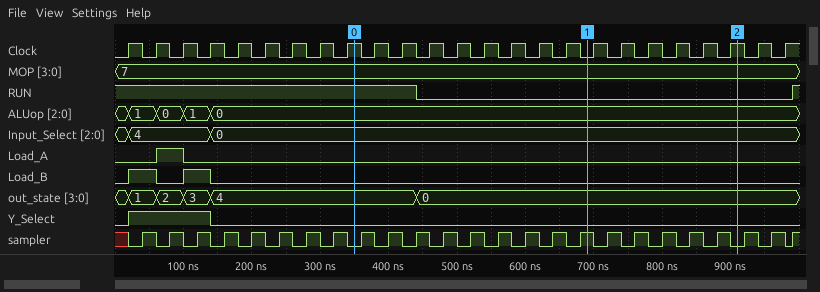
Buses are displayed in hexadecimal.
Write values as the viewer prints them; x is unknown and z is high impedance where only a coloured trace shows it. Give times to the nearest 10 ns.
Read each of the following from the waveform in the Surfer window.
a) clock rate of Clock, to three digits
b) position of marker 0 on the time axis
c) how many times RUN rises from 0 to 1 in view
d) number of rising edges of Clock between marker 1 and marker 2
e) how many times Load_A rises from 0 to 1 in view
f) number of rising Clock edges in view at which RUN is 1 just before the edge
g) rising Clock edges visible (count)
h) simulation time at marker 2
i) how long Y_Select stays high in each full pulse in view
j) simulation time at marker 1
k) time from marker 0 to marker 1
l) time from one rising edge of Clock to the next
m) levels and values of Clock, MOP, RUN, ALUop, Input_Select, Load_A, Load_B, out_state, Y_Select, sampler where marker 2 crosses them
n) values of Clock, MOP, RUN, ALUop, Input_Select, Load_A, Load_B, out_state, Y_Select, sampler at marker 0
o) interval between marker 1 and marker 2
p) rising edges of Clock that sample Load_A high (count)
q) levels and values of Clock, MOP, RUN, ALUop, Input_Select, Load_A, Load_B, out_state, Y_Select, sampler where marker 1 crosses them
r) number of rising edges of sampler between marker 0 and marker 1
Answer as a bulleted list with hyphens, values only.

- 25.0 MHz
- 350 ns
- 1
- 6
- 1
- 11
- 25
- 910 ns
- 120 ns
- 690 ns
- 340 ns
- 40 ns
- Clock=1, MOP=7, RUN=0, ALUop=0, Input_Select=0, Load_A=0, Load_B=0, out_state=0, Y_Select=0, sampler=0
- Clock=1, MOP=7, RUN=1, ALUop=0, Input_Select=0, Load_A=0, Load_B=0, out_state=4, Y_Select=0, sampler=0
- 220 ns
- 1
- Clock=0, MOP=7, RUN=0, ALUop=0, Input_Select=0, Load_A=0, Load_B=0, out_state=0, Y_Select=0, sampler=1
- 9
